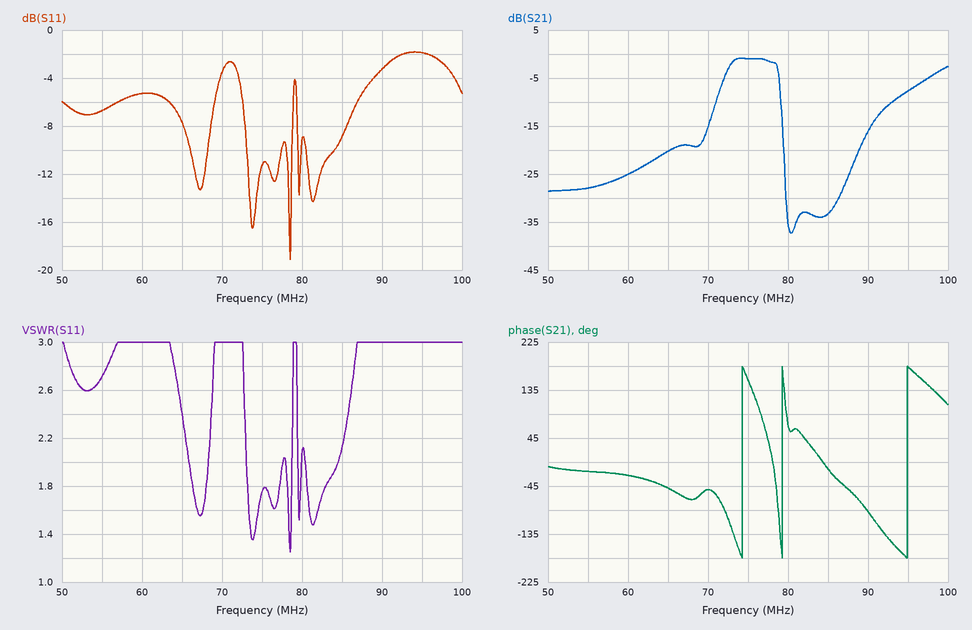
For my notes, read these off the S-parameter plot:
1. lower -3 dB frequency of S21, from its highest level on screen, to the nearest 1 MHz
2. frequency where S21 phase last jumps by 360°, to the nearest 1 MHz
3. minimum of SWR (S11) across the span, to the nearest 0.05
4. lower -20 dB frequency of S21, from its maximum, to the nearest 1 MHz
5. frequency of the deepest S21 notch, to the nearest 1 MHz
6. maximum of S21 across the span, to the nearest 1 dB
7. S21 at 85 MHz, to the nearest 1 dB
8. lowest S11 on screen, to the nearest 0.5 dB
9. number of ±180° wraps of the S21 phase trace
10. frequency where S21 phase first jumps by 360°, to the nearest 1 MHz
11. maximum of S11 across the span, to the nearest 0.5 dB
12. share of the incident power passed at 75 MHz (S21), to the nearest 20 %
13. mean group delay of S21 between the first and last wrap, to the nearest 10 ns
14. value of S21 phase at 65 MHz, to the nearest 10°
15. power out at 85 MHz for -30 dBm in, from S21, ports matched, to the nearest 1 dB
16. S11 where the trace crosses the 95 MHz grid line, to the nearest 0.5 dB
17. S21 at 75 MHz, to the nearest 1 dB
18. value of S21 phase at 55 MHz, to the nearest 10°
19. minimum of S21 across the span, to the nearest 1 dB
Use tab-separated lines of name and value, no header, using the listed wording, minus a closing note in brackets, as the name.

lower -3 dB frequency of S21, from its highest level on screen, to the nearest 1 MHz	72 MHz
frequency where S21 phase last jumps by 360°, to the nearest 1 MHz	95 MHz
minimum of SWR (S11) across the span, to the nearest 0.05	1.25
lower -20 dB frequency of S21, from its maximum, to the nearest 1 MHz	64 MHz
frequency of the deepest S21 notch, to the nearest 1 MHz	80 MHz
maximum of S21 across the span, to the nearest 1 dB	-1 dB
S21 at 85 MHz, to the nearest 1 dB	-33 dB
lowest S11 on screen, to the nearest 0.5 dB	-19.0 dB
number of ±180° wraps of the S21 phase trace	3
frequency where S21 phase first jumps by 360°, to the nearest 1 MHz	74 MHz
maximum of S11 across the span, to the nearest 0.5 dB	-2.0 dB
share of the incident power passed at 75 MHz (S21), to the nearest 20 %	80 %
mean group delay of S21 between the first and last wrap, to the nearest 10 ns	100 ns
value of S21 phase at 65 MHz, to the nearest 10°	-50°
power out at 85 MHz for -30 dBm in, from S21, ports matched, to the nearest 1 dB	-63 dBm
S11 where the trace crosses the 95 MHz grid line, to the nearest 0.5 dB	-2.0 dB
S21 at 75 MHz, to the nearest 1 dB	-1 dB
value of S21 phase at 55 MHz, to the nearest 10°	-20°
minimum of S21 across the span, to the nearest 1 dB	-37 dB
